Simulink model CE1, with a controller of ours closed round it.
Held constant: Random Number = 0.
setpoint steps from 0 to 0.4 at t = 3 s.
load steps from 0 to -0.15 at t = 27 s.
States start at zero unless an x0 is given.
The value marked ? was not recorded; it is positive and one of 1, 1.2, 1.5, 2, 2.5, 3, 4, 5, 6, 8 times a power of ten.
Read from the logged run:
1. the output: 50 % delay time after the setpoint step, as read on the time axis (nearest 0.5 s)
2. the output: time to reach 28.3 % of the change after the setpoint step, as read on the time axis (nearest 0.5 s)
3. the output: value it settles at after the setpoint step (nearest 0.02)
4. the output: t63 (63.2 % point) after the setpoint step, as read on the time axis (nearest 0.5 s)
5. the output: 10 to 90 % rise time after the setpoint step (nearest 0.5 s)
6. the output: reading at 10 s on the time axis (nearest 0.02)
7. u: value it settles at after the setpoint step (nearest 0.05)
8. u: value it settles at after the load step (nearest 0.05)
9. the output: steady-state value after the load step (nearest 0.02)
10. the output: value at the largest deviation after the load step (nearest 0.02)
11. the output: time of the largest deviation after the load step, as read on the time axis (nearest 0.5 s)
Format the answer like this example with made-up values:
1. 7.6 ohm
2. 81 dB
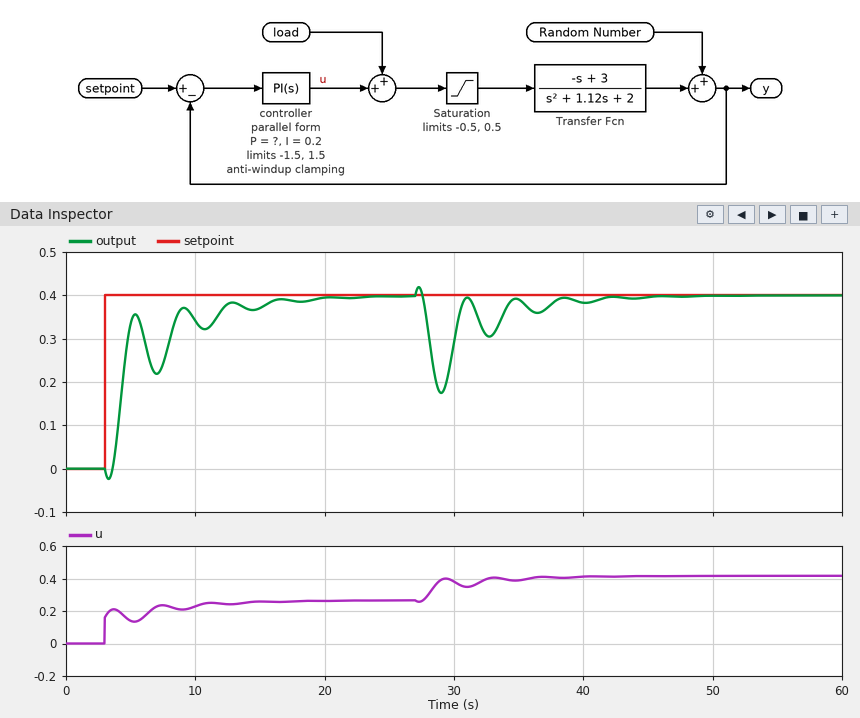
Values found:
1. 4.5 s
2. 4.0 s
3. 0.40
4. 4.5 s
5. 5.0 s
6. 0.34
7. 0.25
8. 0.40
9. 0.40
10. 0.18
11. 29.0 s
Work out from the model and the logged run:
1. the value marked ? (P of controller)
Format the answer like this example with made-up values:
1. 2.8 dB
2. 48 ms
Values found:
1. 0.4
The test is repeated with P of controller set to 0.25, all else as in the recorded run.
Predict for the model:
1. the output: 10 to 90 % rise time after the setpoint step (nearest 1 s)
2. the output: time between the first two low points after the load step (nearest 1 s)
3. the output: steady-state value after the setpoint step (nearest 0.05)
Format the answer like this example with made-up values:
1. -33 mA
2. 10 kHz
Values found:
1. 6 s
2. 4 s
3. 0.40
